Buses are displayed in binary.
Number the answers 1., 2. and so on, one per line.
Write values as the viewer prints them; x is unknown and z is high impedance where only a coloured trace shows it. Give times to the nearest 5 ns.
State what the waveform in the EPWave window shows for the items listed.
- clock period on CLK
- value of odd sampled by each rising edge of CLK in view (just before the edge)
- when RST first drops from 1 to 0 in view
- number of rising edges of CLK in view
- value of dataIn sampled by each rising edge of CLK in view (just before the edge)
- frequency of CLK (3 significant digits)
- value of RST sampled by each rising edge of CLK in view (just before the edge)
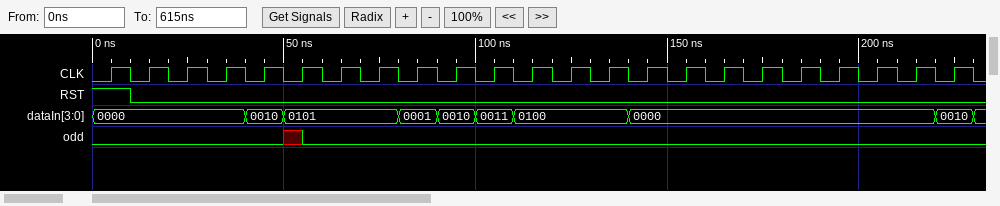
1. 10 ns
2. 0 0 0 0 0 x 0 0 0 0 0 0 0 0 0 0 0 0 0 0 0 0 0
3. 10 ns
4. 23
5. 0000, 0000, 0000, 0000, 0010, 0101, 0101, 0101, 0001, 0010, 0011, 0100, 0100, 0100, 0000, 0000, 0000, 0000, 0000, 0000, 0000, 0000, 0010
6. 100 MHz
7. 1 0 0 0 0 0 0 0 0 0 0 0 0 0 0 0 0 0 0 0 0 0 0
